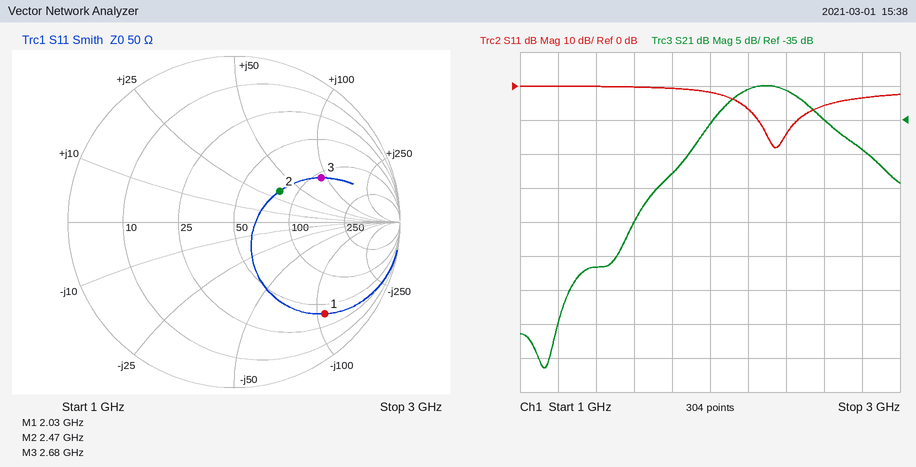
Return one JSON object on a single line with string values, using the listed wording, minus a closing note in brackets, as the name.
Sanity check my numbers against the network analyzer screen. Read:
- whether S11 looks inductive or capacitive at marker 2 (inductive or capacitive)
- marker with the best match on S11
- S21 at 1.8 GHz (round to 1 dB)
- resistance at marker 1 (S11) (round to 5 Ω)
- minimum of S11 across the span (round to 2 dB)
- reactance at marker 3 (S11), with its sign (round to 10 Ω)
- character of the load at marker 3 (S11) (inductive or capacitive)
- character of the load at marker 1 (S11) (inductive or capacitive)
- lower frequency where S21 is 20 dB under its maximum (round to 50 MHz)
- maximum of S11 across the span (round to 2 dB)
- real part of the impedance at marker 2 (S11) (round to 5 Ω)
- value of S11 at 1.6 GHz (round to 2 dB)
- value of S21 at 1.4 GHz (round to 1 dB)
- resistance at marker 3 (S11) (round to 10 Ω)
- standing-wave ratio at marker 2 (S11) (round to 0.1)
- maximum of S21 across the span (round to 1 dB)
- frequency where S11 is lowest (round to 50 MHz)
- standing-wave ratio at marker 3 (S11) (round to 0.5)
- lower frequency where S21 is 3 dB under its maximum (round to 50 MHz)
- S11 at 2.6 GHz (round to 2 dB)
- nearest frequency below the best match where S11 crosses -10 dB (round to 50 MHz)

{"whether S11 looks inductive or capacitive at marker 2": "inductive", "marker with the best match on S11": "marker 2", "S21 at 1.8 GHz": "-43 dB", "resistance at marker 1 (S11)": "40 Ω", "minimum of S11 across the span": "-18 dB", "reactance at marker 3 (S11), with its sign": "+90 Ω", "character of the load at marker 3 (S11)": "inductive", "character of the load at marker 1 (S11)": "capacitive", "lower frequency where S21 is 20 dB under its maximum": "1.60 GHz", "maximum of S11 across the span": "0 dB", "real part of the impedance at marker 2 (S11)": "80 Ω", "value of S11 at 1.6 GHz": "0 dB", "value of S21 at 1.4 GHz": "-57 dB", "resistance at marker 3 (S11)": "110 Ω", "standing-wave ratio at marker 2 (S11)": "2.0", "maximum of S21 across the span": "-30 dB", "frequency where S11 is lowest": "2.35 GHz", "standing-wave ratio at marker 3 (S11)": "4.0", "lower frequency where S21 is 3 dB under its maximum": "2.10 GHz", "S11 at 2.6 GHz": "-6 dB", "nearest frequency below the best match where S11 crosses -10 dB": "2.25 GHz"}
